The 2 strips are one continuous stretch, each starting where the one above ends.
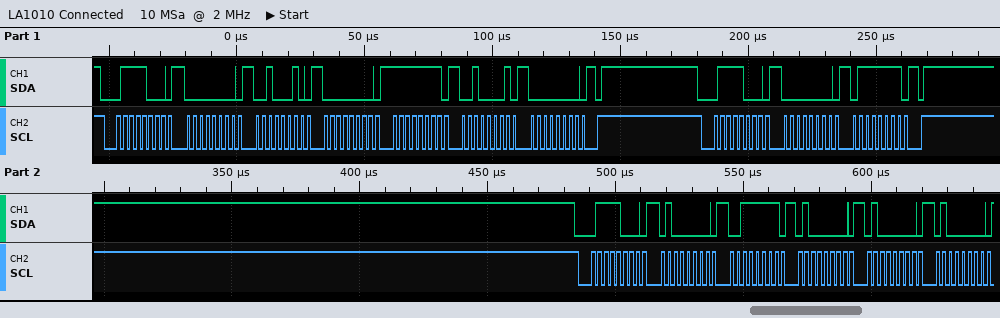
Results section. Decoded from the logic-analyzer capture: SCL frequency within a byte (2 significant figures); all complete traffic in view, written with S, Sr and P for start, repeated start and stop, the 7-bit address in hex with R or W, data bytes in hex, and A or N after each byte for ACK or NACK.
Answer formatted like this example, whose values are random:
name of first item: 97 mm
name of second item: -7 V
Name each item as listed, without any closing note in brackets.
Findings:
SCL frequency within a byte: 400 kHz
all complete traffic in view, written with S, Sr and P for start, repeated start and stop, the 7-bit address in hex with R or W, data bytes in hex, and A or N after each byte for ACK or NACK: S 3CW A 00 A 22 A 00 A FF A 21 A 00 A P S 3CW A 00 A 7F A P S 3CW A 40 A 3F A 40 A 40 A 40 A
